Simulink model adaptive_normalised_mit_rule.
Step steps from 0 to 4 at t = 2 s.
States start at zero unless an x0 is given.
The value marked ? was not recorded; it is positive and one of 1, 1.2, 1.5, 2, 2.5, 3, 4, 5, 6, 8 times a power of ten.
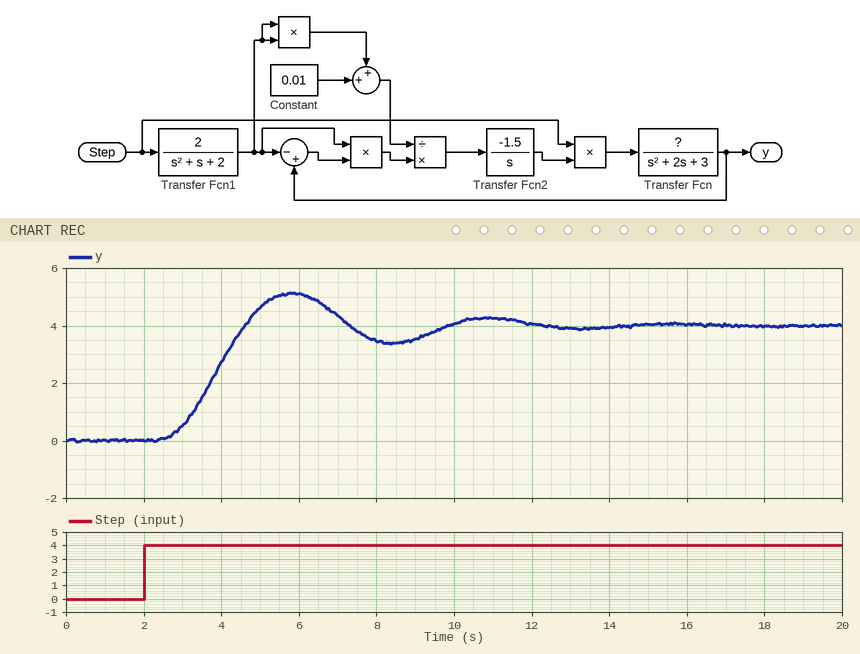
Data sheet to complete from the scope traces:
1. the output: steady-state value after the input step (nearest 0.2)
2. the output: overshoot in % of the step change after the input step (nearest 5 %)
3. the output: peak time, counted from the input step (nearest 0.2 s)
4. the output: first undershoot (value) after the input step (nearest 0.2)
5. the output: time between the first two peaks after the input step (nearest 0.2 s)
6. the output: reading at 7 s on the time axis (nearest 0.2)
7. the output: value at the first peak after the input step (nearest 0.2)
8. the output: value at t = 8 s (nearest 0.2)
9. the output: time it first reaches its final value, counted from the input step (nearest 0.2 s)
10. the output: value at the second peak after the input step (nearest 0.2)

4.0
30 %
3.8 s
3.4
5.0 s
4.4
5.2
3.4
2.6 s
4.2
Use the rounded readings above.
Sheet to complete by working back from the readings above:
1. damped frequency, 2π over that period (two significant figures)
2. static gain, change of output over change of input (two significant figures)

1.3 rad/s
1.0
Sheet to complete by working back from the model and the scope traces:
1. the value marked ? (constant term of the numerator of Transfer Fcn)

1.5
